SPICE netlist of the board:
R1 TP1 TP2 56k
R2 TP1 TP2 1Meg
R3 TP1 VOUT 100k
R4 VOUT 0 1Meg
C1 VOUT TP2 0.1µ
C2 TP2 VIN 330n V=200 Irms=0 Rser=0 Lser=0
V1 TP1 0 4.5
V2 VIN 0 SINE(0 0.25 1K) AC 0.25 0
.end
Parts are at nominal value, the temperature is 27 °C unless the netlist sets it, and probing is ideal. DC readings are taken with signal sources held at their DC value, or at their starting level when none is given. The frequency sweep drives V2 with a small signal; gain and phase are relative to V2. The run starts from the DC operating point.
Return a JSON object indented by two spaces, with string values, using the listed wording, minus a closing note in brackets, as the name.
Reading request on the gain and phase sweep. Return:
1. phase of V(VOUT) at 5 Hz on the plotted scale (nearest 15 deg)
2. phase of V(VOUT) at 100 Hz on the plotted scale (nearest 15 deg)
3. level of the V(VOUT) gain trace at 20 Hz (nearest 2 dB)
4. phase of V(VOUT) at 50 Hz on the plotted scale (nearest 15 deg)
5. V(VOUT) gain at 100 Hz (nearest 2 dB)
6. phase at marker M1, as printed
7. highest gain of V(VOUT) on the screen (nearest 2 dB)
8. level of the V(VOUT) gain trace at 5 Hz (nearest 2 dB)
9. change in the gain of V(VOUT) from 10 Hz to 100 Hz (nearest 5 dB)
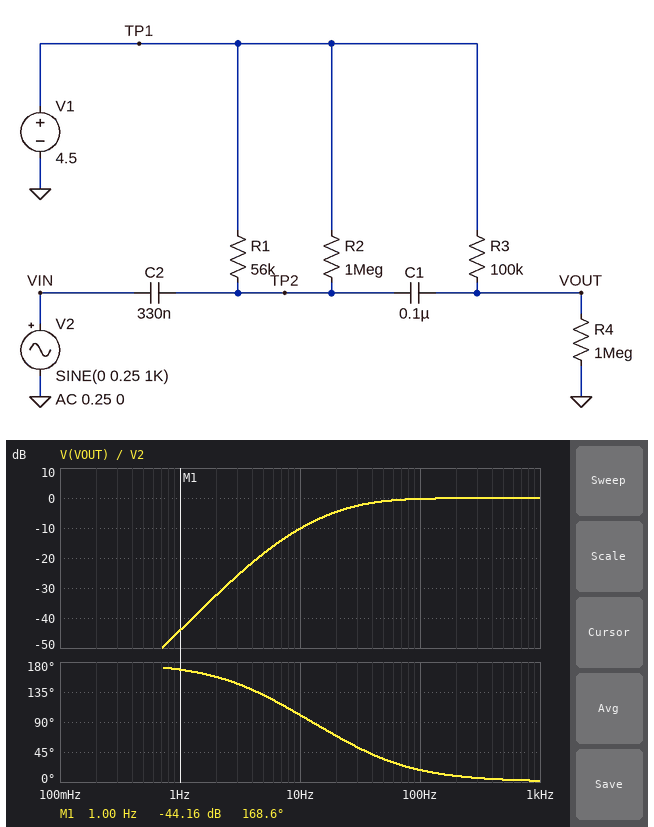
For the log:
{
  "phase of V(VOUT) at 5 Hz on the plotted scale": "135 deg",
  "phase of V(VOUT) at 100 Hz on the plotted scale": "15 deg",
  "level of the V(VOUT) gain trace at 20 Hz": "-4 dB",
  "phase of V(VOUT) at 50 Hz on the plotted scale": "30 deg",
  "V(VOUT) gain at 100 Hz": "0 dB",
  "phase at marker M1, as printed": "168.6 deg",
  "highest gain of V(VOUT) on the screen": "0 dB",
  "level of the V(VOUT) gain trace at 5 Hz": "-18 dB",
  "change in the gain of V(VOUT) from 10 Hz to 100 Hz": "10 dB"
}
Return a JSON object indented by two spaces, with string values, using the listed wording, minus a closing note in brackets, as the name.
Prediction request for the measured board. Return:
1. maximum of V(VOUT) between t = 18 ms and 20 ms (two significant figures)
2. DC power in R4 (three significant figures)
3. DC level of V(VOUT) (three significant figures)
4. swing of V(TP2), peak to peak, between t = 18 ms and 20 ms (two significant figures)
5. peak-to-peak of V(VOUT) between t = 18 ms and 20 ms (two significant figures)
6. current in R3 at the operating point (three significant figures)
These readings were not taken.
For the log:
{
  "maximum of V(VOUT) between t = 18 ms and 20 ms": "4.3 V",
  "DC power in R4": "16.7 µW",
  "DC level of V(VOUT)": "4.09 V",
  "swing of V(TP2), peak to peak, between t = 18 ms and 20 ms": "500 mV",
  "peak-to-peak of V(VOUT) between t = 18 ms and 20 ms": "500 mV",
  "current in R3 at the operating point": "4.09 µA"
}
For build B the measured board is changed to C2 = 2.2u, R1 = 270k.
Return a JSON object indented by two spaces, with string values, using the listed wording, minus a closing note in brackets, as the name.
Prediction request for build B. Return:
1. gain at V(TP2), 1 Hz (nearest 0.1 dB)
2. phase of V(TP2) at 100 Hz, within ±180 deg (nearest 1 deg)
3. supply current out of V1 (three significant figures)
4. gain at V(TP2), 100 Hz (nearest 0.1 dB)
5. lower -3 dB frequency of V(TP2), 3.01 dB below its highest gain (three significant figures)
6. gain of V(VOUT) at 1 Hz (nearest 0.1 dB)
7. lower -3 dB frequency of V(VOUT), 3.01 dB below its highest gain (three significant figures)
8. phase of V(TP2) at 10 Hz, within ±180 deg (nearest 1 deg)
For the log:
{
  "gain at V(TP2), 1 Hz": "-0.8 dB",
  "phase of V(TP2) at 100 Hz, within ±180 deg": "1 deg",
  "supply current out of V1": "4.09 µA",
  "gain at V(TP2), 100 Hz": "0 dB",
  "lower -3 dB frequency of V(TP2), 3.01 dB below its highest gain": "358 mHz",
  "gain of V(VOUT) at 1 Hz": "-25.7 dB",
  "lower -3 dB frequency of V(VOUT), 3.01 dB below its highest gain": "18.3 Hz",
  "phase of V(TP2) at 10 Hz, within ±180 deg": "3 deg"
}
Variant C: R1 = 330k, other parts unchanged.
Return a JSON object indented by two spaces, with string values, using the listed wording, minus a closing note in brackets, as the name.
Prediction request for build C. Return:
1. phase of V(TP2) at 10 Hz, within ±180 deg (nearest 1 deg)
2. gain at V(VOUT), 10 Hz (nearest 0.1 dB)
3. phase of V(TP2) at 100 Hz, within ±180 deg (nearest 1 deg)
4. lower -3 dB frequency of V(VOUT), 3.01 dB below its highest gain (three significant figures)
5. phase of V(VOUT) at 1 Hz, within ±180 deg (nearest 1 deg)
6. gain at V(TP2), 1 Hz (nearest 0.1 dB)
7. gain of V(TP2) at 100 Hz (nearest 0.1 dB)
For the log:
{
  "phase of V(TP2) at 10 Hz, within ±180 deg": "15 deg",
  "gain at V(VOUT), 10 Hz": "-8.2 dB",
  "phase of V(TP2) at 100 Hz, within ±180 deg": "4 deg",
  "lower -3 dB frequency of V(VOUT), 3.01 dB below its highest gain": "23.4 Hz",
  "phase of V(VOUT) at 1 Hz, within ±180 deg": "143 deg",
  "gain at V(TP2), 1 Hz": "-7.4 dB",
  "gain of V(TP2) at 100 Hz": "-0.1 dB"
}
